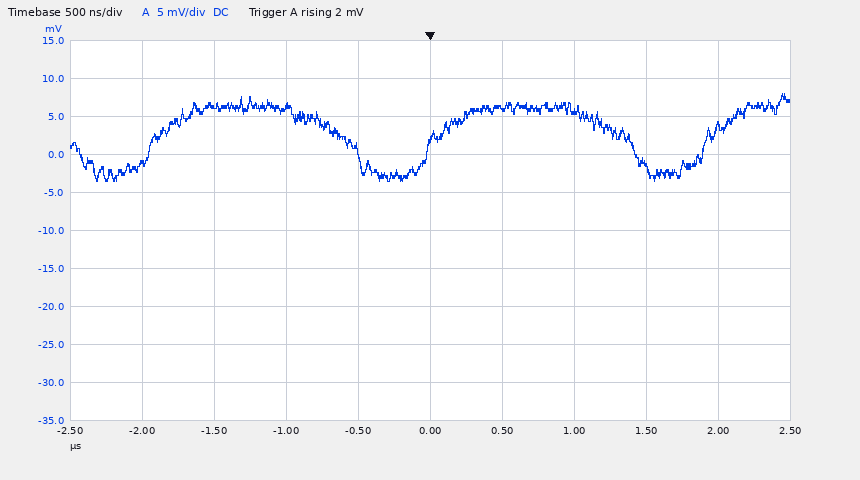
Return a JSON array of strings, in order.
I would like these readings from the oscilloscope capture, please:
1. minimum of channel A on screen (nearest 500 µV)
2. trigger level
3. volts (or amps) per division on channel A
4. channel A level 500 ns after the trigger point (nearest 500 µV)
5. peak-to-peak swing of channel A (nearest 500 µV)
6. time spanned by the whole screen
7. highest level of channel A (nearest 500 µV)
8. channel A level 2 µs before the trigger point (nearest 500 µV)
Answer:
["-3.5 mV", "2 mV", "5 mV", "6.0 mV", "11.5 mV", "5 µs", "8.0 mV", "-1.0 mV"]
